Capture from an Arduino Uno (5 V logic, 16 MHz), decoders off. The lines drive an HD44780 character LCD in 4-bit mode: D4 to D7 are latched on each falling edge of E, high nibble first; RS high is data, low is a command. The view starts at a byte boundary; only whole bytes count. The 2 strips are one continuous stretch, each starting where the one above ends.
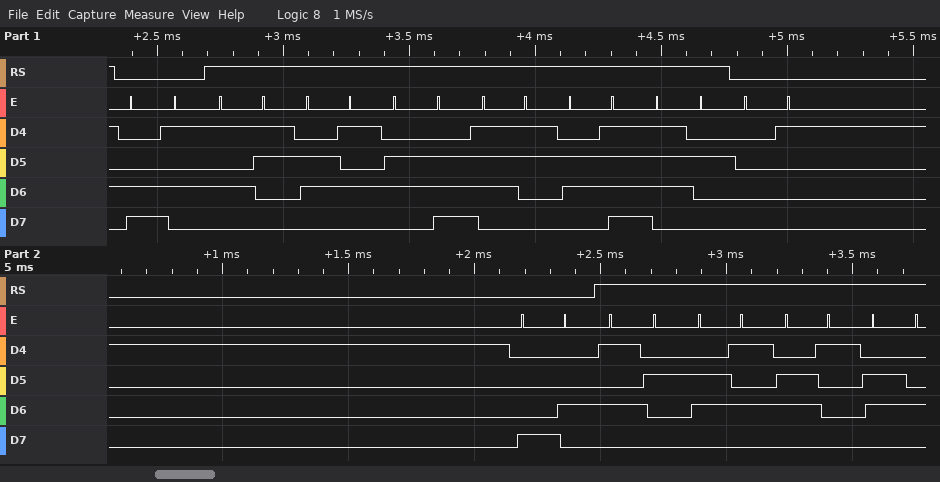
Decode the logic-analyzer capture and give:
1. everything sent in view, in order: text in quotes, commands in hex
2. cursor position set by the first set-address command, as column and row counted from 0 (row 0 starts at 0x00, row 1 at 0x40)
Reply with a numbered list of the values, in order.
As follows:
1. 0xC5 "Sensor" 0x01 0x84 "Read"
2. column 5, row 1
